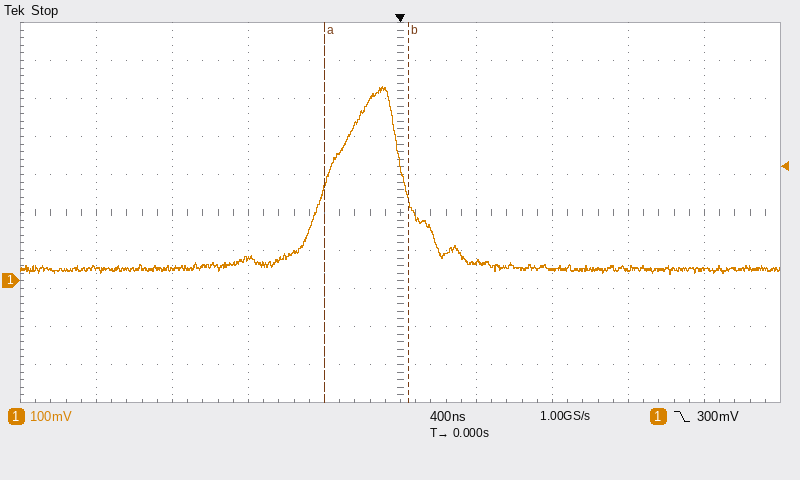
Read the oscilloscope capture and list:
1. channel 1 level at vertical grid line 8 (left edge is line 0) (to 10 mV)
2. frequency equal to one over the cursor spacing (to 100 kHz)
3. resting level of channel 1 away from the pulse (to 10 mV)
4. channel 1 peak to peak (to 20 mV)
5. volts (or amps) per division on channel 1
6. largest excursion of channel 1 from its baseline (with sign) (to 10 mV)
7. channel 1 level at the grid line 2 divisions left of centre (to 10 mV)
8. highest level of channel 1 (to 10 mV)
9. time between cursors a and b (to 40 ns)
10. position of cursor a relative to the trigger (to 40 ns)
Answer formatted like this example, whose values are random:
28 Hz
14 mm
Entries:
30 mV
2.3 MHz
30 mV
500 mV
100 mV
+480 mV
60 mV
510 mV
440 ns
-400 ns
